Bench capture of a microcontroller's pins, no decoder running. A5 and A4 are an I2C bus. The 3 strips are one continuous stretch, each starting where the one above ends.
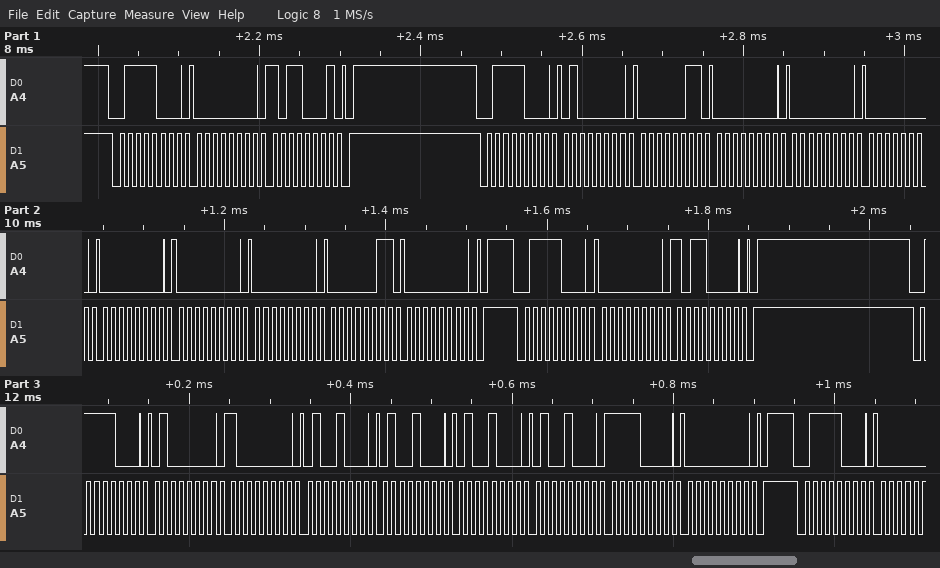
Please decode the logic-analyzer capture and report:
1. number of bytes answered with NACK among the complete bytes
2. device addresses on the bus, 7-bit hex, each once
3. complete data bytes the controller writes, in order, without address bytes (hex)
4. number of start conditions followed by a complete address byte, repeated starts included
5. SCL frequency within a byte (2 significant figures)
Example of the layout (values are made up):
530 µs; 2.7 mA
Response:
0; 0x3C; 00 B1 40 03 00 00 00 00 00 00 03 00 00 B0 40 80 48 48 48 48 F0 00; 5; 100 kHz
